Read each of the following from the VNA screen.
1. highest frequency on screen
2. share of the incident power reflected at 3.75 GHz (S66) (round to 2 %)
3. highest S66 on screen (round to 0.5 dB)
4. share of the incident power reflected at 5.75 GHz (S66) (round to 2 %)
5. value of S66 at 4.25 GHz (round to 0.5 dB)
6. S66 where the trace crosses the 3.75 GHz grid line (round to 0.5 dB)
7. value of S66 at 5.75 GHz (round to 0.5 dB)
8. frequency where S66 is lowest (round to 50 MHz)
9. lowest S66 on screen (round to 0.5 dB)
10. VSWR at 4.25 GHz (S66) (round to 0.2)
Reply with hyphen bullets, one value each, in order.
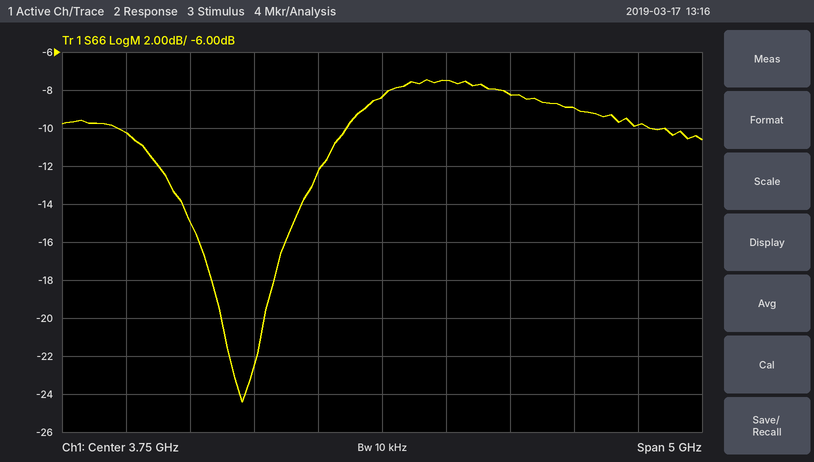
- 6.25 GHz
- 14 %
- -7.5 dB
- 10 %
- -7.5 dB
- -8.5 dB
- -10.0 dB
- 2.65 GHz
- -24.5 dB
- 2.4
